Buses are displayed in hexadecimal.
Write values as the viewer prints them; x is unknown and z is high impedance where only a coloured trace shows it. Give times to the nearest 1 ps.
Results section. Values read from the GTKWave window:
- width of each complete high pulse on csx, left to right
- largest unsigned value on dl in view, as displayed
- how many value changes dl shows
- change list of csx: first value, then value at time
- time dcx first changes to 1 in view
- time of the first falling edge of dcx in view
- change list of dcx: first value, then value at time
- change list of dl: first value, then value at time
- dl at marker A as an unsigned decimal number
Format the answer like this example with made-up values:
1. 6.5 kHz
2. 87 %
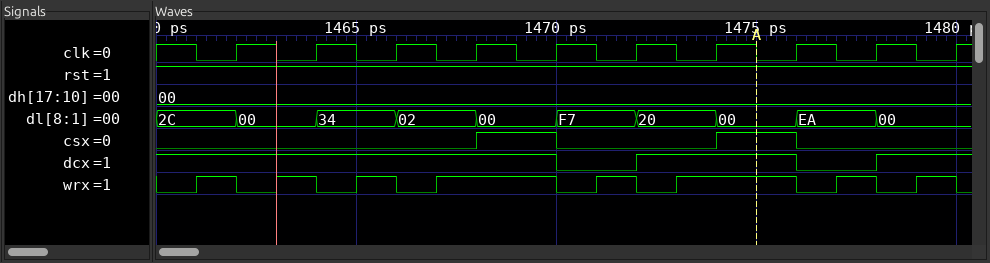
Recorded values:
1. 2 ps, 2 ps
2. F7
3. 9
4. 0, 1 at 1468 ps, 0 at 1470 ps, 1 at 1474 ps, 0 at 1476 ps
5. 1472 ps
6. 1470 ps
7. 1, 0 at 1470 ps, 1 at 1472 ps, 0 at 1476 ps, 1 at 1478 ps
8. 2C, 00 at 1462 ps, 34 at 1464 ps, 02 at 1466 ps, 00 at 1468 ps, F7 at 1470 ps, 20 at 1472 ps, 00 at 1474 ps, EA at 1476 ps, 00 at 1478 ps
9. 0
